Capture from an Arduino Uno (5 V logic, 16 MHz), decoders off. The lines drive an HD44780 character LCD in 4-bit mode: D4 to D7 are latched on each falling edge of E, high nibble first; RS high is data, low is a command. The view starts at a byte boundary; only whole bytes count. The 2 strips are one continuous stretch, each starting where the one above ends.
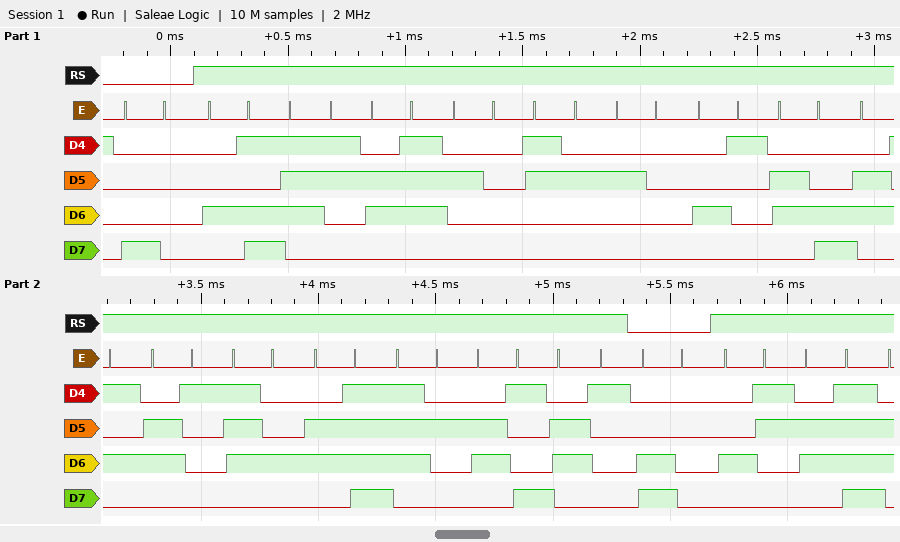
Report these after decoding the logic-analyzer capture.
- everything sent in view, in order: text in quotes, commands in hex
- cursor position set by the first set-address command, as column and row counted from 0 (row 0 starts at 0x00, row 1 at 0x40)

0x80 "Msg 2 Aleatoria" 0xC0 "Co"
column 0, row 0
